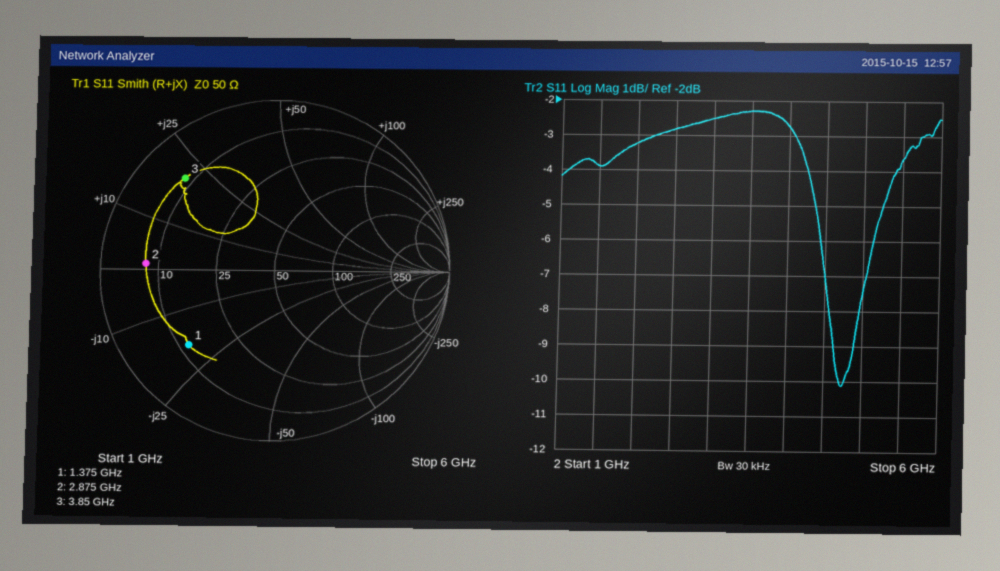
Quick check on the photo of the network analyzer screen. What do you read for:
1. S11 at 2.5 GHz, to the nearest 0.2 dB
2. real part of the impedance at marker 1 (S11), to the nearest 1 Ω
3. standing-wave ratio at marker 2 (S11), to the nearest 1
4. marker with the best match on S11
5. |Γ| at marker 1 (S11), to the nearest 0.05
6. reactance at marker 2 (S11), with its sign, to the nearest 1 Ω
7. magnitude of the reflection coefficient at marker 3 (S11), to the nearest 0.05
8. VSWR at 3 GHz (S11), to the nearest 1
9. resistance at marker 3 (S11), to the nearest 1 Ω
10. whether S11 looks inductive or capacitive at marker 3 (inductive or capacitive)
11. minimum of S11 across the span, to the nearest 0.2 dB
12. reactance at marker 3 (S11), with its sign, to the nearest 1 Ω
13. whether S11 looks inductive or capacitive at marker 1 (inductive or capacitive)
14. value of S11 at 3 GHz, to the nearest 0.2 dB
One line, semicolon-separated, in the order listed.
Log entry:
-2.8 dB; 12 Ω; 7; marker 1; 0.65; +1 Ω; 0.75; 7; 8 Ω; inductive; -10.2 dB; +20 Ω; capacitive; -2.6 dB
